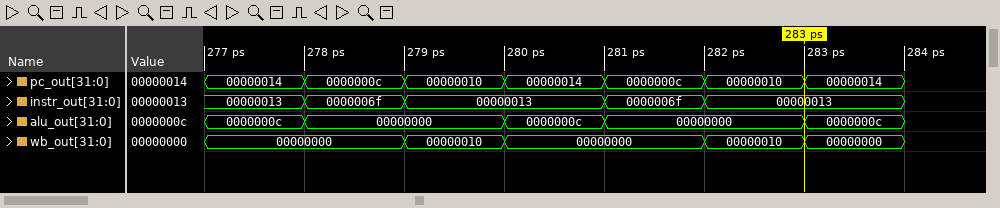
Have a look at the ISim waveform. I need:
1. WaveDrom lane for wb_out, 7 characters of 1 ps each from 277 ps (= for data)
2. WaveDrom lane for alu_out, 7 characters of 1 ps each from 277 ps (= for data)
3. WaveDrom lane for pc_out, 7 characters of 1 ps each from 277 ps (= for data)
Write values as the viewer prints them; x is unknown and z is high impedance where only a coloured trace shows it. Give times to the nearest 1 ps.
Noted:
{name: 'wb_out', wave: '=.==.==', data: '00000000 00000010 00000000 00000010 00000000'}
{name: 'alu_out', wave: '==.==.=', data: '0000000c 00000000 0000000c 00000000 0000000c'}
{name: 'pc_out', wave: '=======', data: '00000014 0000000c 00000010 00000014 0000000c 00000010 00000014'}
